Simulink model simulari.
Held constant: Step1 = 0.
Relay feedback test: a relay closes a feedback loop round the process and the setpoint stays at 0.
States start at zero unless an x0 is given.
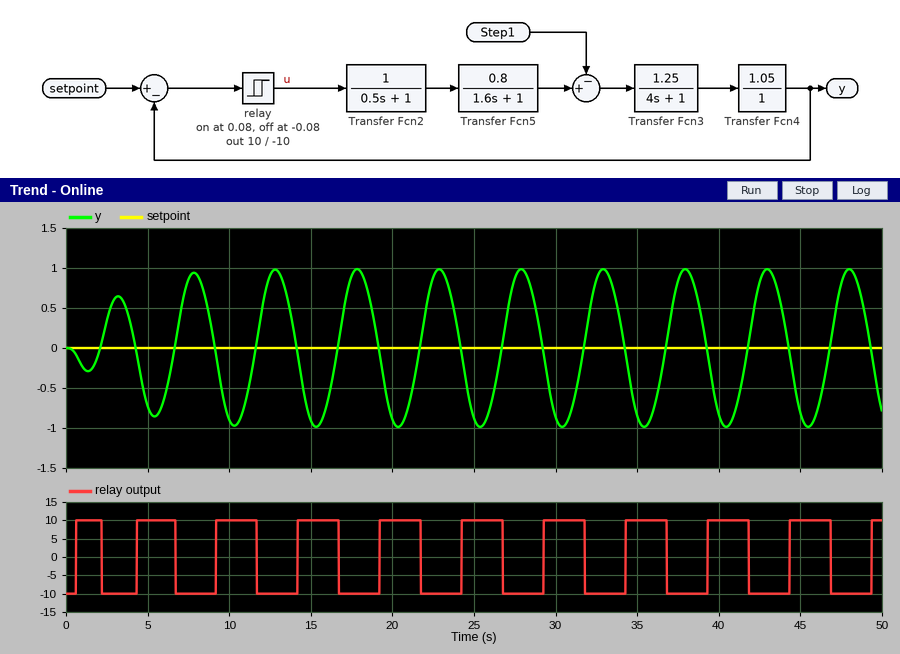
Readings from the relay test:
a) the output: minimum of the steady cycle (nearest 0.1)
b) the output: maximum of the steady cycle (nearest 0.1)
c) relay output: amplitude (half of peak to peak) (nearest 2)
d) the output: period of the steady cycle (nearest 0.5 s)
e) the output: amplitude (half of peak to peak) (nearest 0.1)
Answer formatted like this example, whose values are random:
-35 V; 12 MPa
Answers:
-1.0; 1.0; 10; 5.0 s; 1.0
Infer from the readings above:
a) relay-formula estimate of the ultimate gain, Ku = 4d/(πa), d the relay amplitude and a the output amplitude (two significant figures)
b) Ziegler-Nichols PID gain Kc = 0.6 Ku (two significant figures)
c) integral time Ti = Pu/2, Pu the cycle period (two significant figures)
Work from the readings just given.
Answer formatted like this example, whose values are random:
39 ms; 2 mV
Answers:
13; 7.8; 2.5 s
